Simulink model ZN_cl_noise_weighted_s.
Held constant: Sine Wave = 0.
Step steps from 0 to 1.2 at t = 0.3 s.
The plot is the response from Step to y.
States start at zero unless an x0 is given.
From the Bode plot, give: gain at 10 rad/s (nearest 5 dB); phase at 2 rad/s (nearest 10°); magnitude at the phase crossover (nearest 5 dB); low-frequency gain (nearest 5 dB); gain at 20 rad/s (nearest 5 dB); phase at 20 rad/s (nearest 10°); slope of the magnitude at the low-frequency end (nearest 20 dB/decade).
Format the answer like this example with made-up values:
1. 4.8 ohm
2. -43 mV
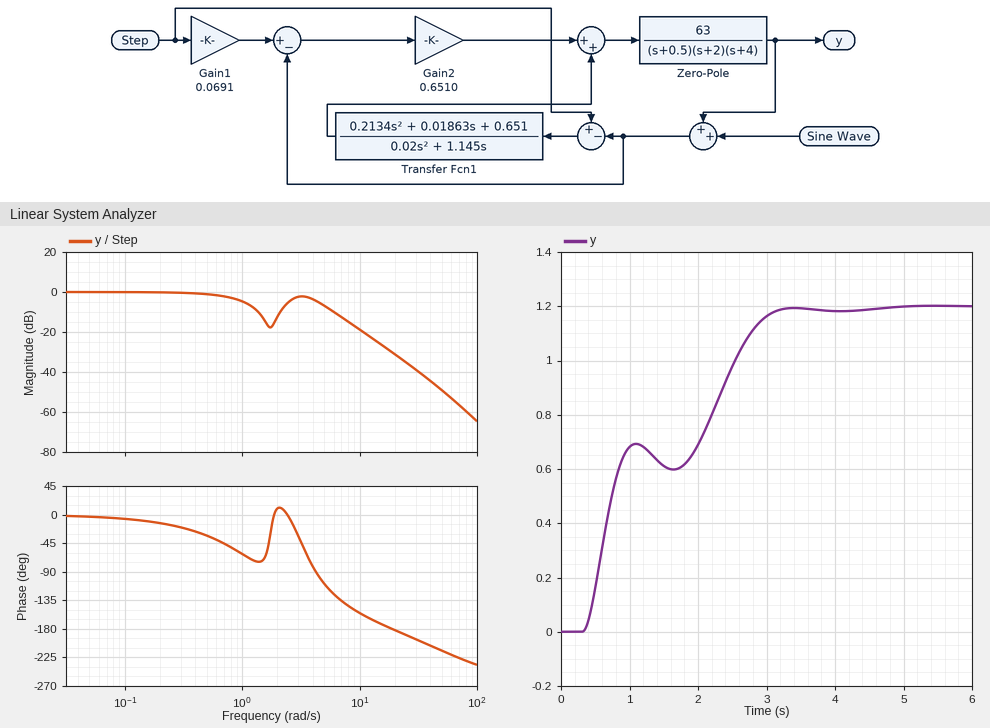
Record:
1. -20 dB
2. 10°
3. -30 dB
4. 0 dB
5. -30 dB
6. -180°
7. 0 dB/decade
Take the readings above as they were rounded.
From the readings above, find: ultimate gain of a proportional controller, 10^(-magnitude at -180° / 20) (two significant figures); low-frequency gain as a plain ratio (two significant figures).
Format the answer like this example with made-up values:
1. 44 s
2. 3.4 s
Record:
1. 32
2. 1.0
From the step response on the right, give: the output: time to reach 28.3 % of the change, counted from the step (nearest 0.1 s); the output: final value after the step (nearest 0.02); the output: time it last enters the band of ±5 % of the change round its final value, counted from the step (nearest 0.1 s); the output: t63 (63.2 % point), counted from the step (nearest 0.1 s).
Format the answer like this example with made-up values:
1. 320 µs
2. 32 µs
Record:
1. 0.3 s
2. 1.20
3. 2.6 s
4. 1.8 s
